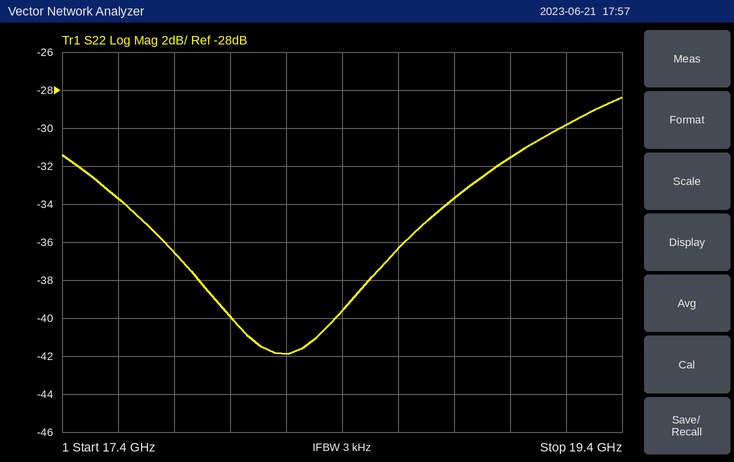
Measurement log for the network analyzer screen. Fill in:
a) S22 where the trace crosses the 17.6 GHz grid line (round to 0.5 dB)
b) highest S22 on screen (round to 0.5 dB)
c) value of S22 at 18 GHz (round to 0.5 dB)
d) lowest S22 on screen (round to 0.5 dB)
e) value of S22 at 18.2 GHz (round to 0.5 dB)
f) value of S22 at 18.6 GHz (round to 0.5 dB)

-33.5 dB
-28.5 dB
-40.0 dB
-42.0 dB
-42.0 dB
-36.5 dB
